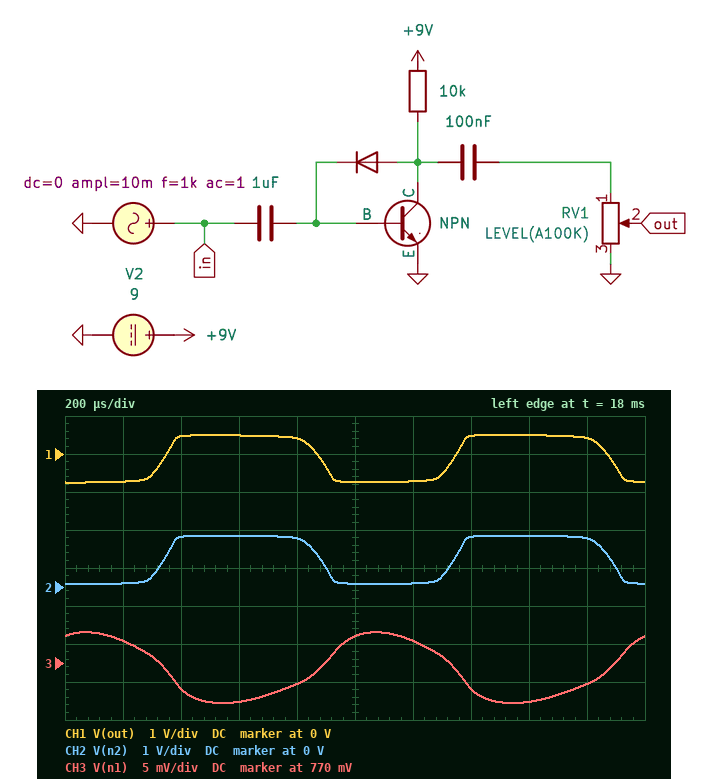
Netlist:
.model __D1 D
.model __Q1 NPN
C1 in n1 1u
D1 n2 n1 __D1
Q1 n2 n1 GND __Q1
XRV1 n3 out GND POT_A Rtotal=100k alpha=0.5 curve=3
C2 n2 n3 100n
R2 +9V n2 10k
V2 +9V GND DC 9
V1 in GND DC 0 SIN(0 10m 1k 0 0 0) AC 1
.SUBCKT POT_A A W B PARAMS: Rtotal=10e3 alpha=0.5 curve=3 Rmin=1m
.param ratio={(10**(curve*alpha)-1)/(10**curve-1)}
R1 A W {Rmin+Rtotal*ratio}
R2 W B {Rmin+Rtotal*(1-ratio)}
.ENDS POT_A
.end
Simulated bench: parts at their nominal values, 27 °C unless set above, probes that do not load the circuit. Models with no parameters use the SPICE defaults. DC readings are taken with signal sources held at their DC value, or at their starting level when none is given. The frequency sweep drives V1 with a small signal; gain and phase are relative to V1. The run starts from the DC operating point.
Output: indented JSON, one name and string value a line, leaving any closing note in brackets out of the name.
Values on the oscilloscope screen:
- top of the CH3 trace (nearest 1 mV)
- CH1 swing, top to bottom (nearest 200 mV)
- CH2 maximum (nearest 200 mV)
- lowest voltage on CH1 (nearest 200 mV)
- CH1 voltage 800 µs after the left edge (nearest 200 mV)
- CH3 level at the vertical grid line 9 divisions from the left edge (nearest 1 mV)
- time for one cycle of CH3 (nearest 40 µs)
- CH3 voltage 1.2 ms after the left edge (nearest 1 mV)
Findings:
{
  "top of the CH3 trace": "774 mV",
  "CH1 swing, top to bottom": "1.2 V",
  "CH2 maximum": "1.4 V",
  "lowest voltage on CH1": "-800 mV",
  "CH1 voltage 800 µs after the left edge": "400 mV",
  "CH3 level at the vertical grid line 9 divisions from the left edge": "767 mV",
  "time for one cycle of CH3": "1.00 ms",
  "CH3 voltage 1.2 ms after the left edge": "773 mV"
}
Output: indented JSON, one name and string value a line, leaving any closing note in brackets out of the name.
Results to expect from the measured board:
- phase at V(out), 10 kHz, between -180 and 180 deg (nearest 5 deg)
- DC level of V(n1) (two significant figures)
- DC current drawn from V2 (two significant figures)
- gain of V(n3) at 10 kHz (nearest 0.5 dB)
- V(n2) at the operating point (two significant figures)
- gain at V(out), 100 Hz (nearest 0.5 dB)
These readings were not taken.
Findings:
{
  "phase at V(out), 10 kHz, between -180 and 180 deg": "-160 deg",
  "DC level of V(n1)": "770 mV",
  "DC current drawn from V2": "770 µA",
  "gain of V(n3) at 10 kHz": "36.5 dB",
  "V(n2) at the operating point": "1.3 V",
  "gain at V(out), 100 Hz": "6.0 dB"
}
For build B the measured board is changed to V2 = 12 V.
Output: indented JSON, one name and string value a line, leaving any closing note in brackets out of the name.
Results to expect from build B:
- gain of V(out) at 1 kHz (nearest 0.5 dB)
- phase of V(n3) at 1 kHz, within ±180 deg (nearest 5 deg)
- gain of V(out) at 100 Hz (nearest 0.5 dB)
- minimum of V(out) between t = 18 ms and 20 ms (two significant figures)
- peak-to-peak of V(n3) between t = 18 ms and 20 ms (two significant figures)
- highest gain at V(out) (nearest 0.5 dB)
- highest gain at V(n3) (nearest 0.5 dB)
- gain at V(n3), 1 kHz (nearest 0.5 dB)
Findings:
{
  "gain of V(out) at 1 kHz": "23.0 dB",
  "phase of V(n3) at 1 kHz, within ±180 deg": "-100 deg",
  "gain of V(out) at 100 Hz": "3.0 dB",
  "minimum of V(out) between t = 18 ms and 20 ms": "-770 mV",
  "peak-to-peak of V(n3) between t = 18 ms and 20 ms": "1.3 V",
  "highest gain at V(out)": "37.5 dB",
  "highest gain at V(n3)": "38.0 dB",
  "gain at V(n3), 1 kHz": "23.5 dB"
}
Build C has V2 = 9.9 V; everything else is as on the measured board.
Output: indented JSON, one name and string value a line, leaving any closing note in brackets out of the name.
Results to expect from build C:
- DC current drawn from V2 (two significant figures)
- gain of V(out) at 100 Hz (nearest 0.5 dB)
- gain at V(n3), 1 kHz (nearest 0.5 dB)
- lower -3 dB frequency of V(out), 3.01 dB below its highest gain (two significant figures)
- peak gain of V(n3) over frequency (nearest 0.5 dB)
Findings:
{
  "DC current drawn from V2": "860 µA",
  "gain of V(out) at 100 Hz": "5.0 dB",
  "gain at V(n3), 1 kHz": "25.0 dB",
  "lower -3 dB frequency of V(out), 3.01 dB below its highest gain": "4.0 kHz",
  "peak gain of V(n3) over frequency": "37.5 dB"
}
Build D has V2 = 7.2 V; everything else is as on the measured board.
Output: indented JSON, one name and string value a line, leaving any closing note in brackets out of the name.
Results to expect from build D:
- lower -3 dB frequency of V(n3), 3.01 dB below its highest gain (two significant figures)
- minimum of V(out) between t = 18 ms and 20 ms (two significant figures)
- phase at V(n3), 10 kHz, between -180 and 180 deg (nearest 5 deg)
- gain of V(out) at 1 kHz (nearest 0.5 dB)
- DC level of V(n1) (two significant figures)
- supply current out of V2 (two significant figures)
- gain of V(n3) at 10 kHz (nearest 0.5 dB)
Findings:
{
  "lower -3 dB frequency of V(n3), 3.01 dB below its highest gain": "2.5 kHz",
  "minimum of V(out) between t = 18 ms and 20 ms": "-740 mV",
  "phase at V(n3), 10 kHz, between -180 and 180 deg": "-165 deg",
  "gain of V(out) at 1 kHz": "27.5 dB",
  "DC level of V(n1)": "760 mV",
  "supply current out of V2": "590 µA",
  "gain of V(n3) at 10 kHz": "36.0 dB"
}
